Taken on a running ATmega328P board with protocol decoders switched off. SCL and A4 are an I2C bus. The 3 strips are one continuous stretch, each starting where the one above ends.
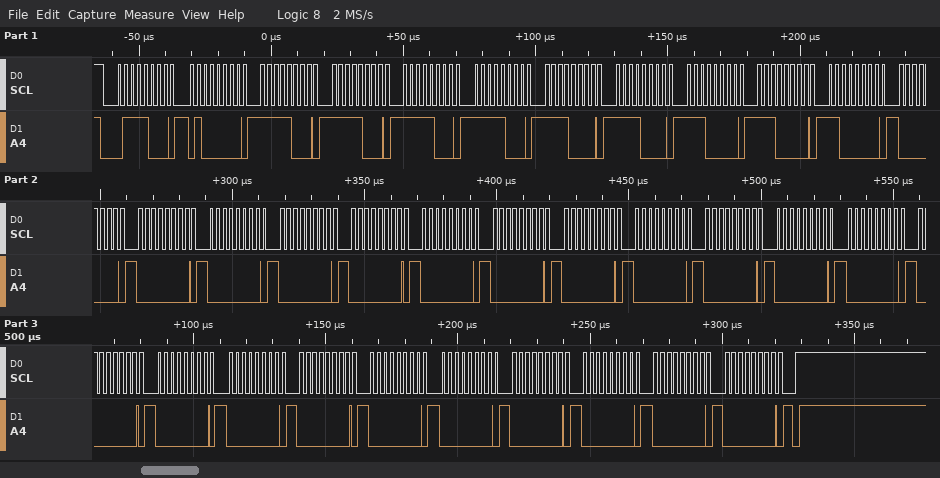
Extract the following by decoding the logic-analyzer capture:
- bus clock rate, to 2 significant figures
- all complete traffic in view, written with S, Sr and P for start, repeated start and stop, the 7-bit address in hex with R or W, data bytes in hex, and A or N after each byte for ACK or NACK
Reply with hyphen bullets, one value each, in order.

- 400 kHz
- S 3CW A 40 A F8 A F8 A F8 A F8 A F0 A F0 A E0 A E0 A C0 A 00 A 00 A 00 A 00 A 00 A 00 A 00 A 00 A 00 A 00 A 00 A 00 A 00 A 00 A 00 A 00 A 00 A 00 A 00 A 00 A 00 A 00 A P
